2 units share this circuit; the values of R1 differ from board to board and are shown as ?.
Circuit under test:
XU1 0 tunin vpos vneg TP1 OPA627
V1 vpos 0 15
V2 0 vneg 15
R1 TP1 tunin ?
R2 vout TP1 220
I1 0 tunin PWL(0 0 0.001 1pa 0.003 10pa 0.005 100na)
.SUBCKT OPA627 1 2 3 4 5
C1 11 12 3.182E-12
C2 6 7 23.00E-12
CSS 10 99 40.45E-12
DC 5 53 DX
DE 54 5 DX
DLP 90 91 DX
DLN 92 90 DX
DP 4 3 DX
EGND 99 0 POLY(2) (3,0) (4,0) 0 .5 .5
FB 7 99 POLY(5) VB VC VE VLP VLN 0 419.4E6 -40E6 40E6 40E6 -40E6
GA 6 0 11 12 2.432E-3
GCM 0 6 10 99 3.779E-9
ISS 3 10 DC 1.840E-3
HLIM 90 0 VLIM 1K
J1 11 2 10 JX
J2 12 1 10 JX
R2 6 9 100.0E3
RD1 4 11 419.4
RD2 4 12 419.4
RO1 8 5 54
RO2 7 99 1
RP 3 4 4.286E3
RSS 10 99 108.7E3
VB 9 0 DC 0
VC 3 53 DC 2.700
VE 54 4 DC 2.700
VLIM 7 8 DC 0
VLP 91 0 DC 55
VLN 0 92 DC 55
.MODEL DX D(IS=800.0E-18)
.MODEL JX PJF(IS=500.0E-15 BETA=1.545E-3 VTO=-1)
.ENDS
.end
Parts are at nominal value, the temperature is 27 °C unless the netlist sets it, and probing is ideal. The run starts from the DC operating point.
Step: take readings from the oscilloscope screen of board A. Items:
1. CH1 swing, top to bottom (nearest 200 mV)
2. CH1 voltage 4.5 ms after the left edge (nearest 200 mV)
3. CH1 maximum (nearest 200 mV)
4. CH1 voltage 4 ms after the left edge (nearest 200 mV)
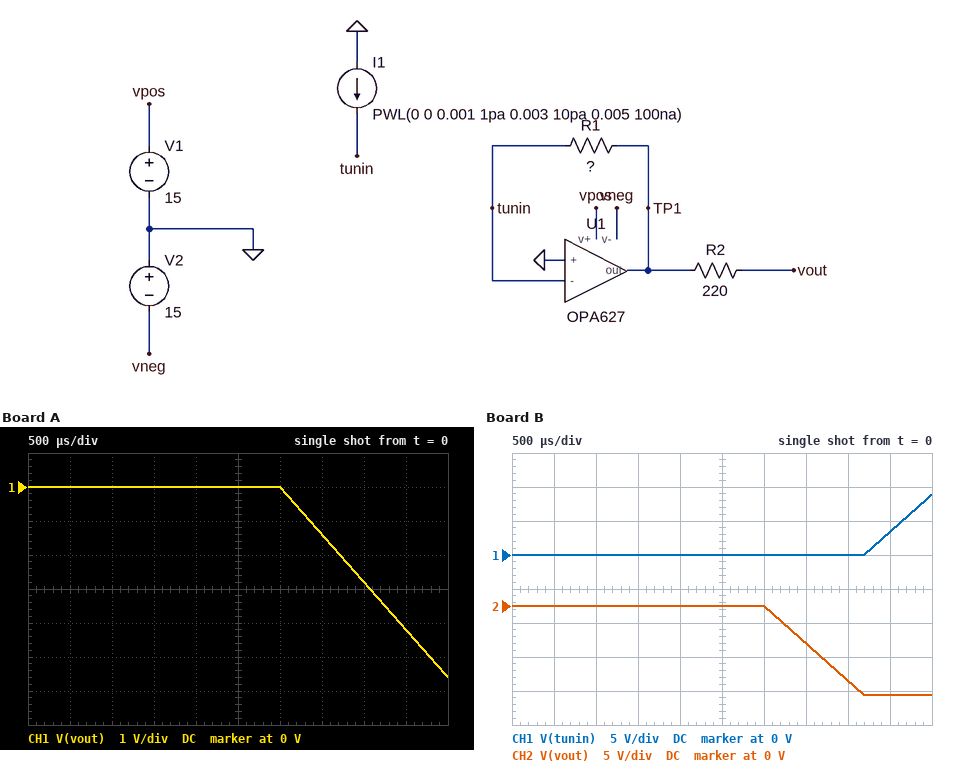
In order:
5.6 V
-4.2 V
0 V
-2.8 V
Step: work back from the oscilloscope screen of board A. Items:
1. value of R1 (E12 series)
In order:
56 MΩ
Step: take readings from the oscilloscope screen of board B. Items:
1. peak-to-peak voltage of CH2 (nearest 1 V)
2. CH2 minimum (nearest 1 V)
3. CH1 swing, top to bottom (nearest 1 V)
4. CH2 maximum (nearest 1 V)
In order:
13 V
-13 V
9 V
0 V
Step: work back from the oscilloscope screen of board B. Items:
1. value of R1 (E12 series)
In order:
220 MΩ
